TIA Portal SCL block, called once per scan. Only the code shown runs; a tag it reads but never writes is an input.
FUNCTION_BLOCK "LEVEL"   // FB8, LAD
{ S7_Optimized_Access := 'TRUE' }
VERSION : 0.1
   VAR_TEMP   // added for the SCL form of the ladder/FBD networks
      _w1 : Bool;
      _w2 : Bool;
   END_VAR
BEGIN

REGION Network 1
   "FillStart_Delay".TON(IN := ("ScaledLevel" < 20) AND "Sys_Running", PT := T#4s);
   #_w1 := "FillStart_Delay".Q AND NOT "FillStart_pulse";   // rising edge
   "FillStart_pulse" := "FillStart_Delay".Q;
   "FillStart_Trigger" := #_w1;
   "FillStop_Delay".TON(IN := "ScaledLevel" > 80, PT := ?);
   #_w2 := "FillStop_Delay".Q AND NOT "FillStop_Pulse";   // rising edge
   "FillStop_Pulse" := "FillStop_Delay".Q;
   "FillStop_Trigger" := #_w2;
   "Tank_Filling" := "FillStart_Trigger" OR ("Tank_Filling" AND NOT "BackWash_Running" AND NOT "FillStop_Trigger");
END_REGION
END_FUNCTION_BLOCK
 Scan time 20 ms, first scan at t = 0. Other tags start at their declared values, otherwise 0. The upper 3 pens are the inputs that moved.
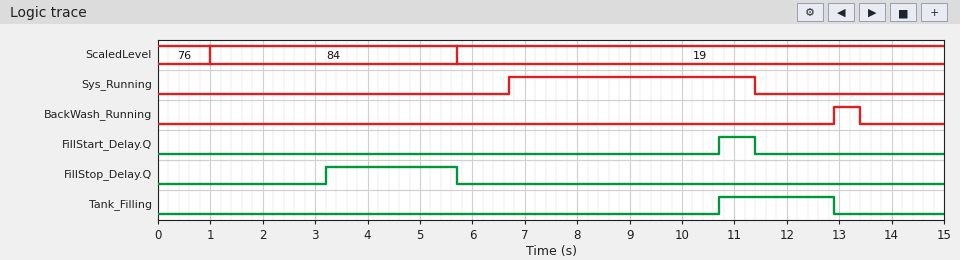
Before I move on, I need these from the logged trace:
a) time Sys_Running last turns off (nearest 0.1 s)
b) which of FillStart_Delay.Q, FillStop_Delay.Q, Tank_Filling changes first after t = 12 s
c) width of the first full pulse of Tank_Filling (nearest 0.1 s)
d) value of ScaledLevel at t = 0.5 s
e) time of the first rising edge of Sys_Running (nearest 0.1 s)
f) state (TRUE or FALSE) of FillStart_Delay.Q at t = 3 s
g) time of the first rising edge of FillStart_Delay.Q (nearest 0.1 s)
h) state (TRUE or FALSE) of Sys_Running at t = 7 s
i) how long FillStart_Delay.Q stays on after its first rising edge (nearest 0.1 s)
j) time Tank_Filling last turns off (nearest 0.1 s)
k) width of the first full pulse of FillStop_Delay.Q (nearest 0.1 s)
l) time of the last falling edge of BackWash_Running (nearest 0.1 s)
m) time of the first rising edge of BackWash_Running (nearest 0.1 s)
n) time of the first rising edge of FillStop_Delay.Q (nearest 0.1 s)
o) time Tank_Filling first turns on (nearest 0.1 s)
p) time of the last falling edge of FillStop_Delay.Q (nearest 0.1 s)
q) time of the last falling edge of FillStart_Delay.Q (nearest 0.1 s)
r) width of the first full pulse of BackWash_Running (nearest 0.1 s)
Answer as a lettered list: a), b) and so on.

a) 11.4 s
b) Tank_Filling
c) 2.2 s
d) 76
e) 6.7 s
f) FALSE
g) 10.7 s
h) TRUE
i) 0.7 s
j) 12.9 s
k) 2.5 s
l) 13.4 s
m) 12.9 s
n) 3.2 s
o) 10.7 s
p) 5.7 s
q) 11.4 s
r) 0.5 s
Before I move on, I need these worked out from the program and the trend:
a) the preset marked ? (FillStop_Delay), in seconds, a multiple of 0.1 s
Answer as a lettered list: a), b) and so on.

a) 2.2 s
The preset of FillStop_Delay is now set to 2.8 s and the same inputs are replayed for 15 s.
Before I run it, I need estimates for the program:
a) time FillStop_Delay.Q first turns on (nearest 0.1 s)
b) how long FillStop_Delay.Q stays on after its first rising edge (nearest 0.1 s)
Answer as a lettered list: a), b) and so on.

a) 3.8 s
b) 1.9 s
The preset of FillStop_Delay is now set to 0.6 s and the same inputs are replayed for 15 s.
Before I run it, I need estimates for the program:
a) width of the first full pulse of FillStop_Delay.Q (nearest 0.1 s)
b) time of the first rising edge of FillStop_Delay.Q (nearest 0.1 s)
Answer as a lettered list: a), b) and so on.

a) 4.1 s
b) 1.6 s
